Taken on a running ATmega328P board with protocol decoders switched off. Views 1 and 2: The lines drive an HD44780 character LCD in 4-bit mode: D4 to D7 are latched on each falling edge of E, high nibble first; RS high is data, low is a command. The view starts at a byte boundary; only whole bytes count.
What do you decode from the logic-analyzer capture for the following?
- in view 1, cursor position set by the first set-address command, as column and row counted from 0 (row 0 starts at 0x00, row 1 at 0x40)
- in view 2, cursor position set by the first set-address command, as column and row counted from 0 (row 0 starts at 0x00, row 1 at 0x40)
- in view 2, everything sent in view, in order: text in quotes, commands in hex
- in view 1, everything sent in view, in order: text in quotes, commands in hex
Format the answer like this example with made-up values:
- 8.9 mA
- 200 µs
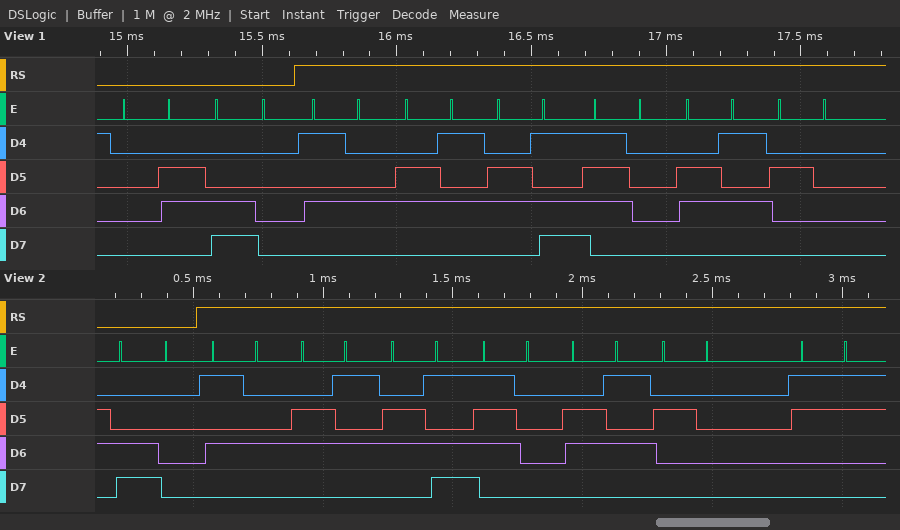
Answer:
- column 0, row 1
- column 0, row 1
- 0xC0 "Tempe 3"
- 0x06 0xC0 "Tempe "
